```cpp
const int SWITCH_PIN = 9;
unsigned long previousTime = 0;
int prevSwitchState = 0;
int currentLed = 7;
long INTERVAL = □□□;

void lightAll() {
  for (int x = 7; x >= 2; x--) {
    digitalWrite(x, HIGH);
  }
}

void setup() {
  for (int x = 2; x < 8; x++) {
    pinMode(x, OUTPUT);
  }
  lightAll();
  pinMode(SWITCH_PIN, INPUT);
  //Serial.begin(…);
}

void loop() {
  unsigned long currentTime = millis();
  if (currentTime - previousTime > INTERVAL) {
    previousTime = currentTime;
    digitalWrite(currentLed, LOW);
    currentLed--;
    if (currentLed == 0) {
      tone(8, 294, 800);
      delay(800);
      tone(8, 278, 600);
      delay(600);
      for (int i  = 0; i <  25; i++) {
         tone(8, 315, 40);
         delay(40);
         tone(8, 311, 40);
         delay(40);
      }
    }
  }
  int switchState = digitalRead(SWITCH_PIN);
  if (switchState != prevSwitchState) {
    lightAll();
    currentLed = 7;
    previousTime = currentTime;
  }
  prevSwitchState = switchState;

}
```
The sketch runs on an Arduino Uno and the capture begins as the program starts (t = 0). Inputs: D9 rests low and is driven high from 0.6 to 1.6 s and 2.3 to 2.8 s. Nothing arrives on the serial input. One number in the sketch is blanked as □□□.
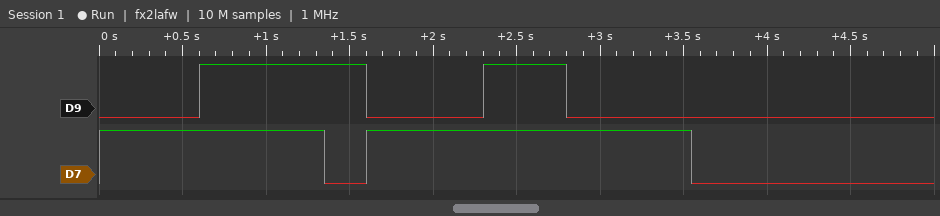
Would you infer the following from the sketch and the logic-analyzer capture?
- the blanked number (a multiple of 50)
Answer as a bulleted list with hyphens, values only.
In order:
- 750
